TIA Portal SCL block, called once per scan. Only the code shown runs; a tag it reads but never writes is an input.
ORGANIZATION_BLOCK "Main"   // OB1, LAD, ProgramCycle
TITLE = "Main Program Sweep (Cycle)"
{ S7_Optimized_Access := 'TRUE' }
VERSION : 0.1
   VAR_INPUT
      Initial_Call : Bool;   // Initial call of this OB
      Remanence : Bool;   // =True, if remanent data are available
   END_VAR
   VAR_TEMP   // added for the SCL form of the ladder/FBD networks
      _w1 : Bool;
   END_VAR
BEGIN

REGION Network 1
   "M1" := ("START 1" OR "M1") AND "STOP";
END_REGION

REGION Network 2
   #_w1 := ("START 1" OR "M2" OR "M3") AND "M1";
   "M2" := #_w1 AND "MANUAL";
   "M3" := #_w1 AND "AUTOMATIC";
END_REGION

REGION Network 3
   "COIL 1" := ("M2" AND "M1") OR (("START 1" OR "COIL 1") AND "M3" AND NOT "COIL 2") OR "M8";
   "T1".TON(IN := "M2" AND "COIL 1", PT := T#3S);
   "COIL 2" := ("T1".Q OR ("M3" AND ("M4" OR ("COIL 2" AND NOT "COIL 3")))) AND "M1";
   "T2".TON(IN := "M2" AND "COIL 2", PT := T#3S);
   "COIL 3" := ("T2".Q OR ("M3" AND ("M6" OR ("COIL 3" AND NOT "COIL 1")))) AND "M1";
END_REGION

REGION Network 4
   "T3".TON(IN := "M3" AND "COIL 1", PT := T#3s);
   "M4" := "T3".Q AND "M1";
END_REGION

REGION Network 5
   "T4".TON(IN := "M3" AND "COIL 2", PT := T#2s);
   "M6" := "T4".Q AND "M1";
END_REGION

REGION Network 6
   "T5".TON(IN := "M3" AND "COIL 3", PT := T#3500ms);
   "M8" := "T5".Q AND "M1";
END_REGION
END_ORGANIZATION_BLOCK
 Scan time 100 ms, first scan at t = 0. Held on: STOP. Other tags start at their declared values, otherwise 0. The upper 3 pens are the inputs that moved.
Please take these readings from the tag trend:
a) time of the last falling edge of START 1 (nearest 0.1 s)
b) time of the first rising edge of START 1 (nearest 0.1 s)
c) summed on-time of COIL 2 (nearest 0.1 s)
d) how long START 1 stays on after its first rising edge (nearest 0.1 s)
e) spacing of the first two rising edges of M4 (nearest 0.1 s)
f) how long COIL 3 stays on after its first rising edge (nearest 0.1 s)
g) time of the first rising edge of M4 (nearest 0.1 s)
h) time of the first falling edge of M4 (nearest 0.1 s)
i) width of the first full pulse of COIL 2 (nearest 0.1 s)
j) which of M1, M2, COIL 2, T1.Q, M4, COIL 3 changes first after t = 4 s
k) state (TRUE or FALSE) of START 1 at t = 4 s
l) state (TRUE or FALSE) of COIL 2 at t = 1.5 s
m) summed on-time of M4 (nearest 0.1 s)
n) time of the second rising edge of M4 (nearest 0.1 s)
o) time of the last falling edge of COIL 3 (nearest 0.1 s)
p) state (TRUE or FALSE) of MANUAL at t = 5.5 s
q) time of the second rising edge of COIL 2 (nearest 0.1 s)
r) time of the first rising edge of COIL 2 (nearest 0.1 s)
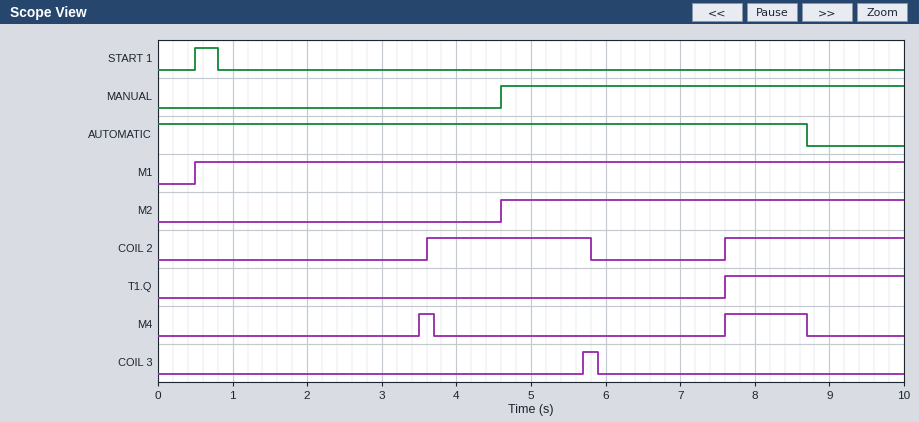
0.8 s
0.5 s
4.6 s
0.3 s
4.1 s
0.2 s
3.5 s
3.7 s
2.2 s
M2
FALSE
FALSE
1.3 s
7.6 s
5.9 s
TRUE
7.6 s
3.6 s
